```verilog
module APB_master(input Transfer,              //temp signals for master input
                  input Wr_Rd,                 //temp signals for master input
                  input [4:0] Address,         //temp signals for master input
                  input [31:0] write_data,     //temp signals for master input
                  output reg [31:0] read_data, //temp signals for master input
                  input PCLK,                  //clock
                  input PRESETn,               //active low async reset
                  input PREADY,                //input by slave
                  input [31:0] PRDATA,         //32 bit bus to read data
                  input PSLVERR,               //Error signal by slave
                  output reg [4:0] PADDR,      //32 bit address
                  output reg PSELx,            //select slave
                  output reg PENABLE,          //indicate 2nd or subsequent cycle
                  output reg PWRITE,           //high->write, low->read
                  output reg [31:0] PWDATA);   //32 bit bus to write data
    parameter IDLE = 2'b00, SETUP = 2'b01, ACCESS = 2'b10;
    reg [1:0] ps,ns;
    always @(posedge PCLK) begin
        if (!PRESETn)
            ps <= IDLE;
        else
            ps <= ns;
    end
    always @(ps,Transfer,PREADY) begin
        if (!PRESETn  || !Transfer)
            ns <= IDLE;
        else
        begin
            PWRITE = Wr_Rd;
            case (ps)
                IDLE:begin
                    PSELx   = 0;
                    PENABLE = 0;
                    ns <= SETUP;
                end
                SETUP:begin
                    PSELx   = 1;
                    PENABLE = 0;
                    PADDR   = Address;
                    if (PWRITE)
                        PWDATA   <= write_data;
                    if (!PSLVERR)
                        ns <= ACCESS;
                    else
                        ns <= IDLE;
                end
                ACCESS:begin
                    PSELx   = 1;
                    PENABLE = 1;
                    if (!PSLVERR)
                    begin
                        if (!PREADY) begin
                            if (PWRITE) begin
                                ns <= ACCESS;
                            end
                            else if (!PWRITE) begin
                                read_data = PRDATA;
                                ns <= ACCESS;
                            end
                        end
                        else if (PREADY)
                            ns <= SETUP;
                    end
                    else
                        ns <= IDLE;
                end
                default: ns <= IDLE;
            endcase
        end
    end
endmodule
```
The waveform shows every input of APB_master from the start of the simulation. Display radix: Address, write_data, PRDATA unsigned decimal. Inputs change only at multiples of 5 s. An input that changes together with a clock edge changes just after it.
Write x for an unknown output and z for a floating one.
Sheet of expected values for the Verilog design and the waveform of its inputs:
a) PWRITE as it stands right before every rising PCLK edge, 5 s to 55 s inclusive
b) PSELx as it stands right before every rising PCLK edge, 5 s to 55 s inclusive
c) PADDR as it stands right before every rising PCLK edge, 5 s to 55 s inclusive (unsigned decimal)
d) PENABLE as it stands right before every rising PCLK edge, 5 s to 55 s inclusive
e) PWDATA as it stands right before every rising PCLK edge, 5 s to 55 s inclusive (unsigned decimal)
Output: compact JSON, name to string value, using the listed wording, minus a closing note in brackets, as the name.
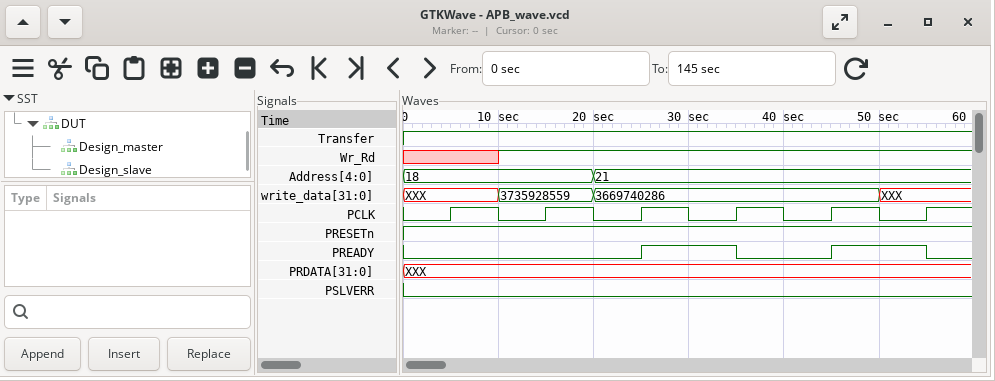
{"PWRITE as it stands right before every rising PCLK edge, 5 s to 55 s inclusive": "x x 1 1 1 1", "PSELx as it stands right before every rising PCLK edge, 5 s to 55 s inclusive": "x 0 1 1 1 1", "PADDR as it stands right before every rising PCLK edge, 5 s to 55 s inclusive": "x, x, 18, 18, 21, 21", "PENABLE as it stands right before every rising PCLK edge, 5 s to 55 s inclusive": "x 0 0 1 0 1", "PWDATA as it stands right before every rising PCLK edge, 5 s to 55 s inclusive": "x, x, 3735928559, 3735928559, 3669740286, 3669740286"}
